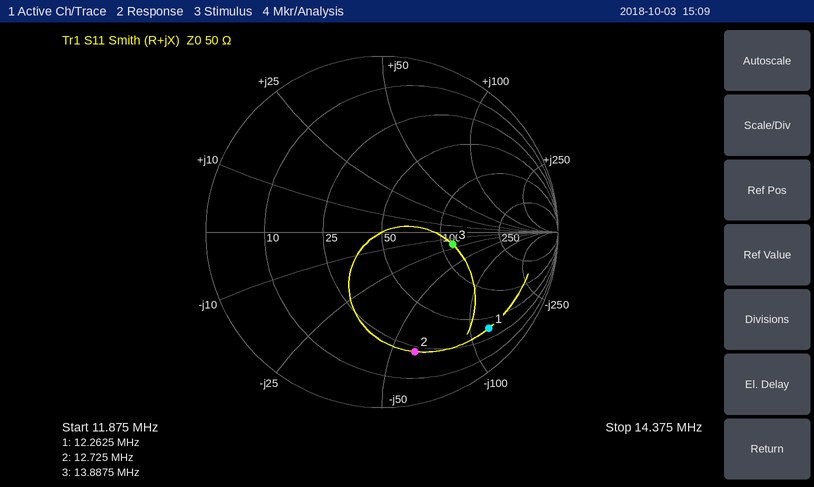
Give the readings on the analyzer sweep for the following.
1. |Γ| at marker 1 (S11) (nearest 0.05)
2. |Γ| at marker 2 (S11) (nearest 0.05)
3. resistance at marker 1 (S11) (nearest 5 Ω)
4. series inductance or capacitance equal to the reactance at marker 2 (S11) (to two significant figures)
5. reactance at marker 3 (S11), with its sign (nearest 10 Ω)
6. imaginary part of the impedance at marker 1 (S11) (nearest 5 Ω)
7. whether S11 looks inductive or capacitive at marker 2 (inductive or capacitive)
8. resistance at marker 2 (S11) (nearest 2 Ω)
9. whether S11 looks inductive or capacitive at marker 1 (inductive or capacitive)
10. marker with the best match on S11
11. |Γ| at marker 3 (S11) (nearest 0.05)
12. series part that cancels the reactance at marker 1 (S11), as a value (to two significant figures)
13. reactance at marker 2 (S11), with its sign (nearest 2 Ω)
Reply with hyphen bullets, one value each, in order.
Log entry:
- 0.80
- 0.70
- 35 Ω
- 210 pF
- -20 Ω
- -120 Ω
- capacitive
- 22 Ω
- capacitive
- marker 3
- 0.40
- 1.6 µH
- -60 Ω
